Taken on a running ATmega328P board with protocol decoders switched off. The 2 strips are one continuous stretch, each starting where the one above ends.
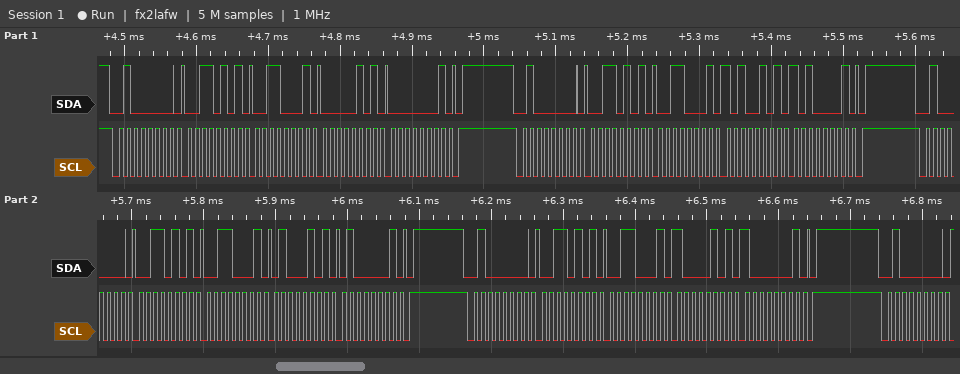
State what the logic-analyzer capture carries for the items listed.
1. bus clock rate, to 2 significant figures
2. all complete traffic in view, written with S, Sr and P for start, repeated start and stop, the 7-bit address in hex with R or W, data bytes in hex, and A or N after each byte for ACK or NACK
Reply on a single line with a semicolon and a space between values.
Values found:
100 kHz; S 20W A 35 A 31 A 05 A 01 A P S 20W A 35 A 31 A A5 A A1 A P S 20W A 35 A 31 A 45 A 41 A P S 20W A 35 A 31 A 85 A 81 A P S 20W A
